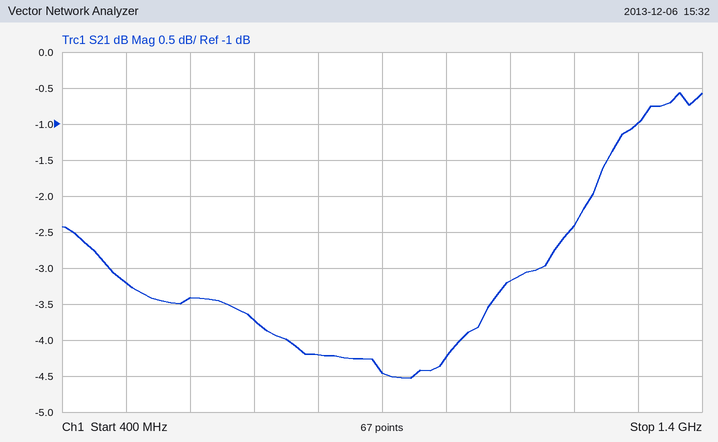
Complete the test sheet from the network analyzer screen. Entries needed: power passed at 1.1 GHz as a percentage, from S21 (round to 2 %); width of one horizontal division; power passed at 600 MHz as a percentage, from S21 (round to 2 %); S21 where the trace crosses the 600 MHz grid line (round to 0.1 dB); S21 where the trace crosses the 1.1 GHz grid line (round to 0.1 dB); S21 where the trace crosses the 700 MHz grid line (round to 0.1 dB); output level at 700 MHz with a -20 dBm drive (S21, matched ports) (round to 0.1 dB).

48 %
100 MHz
46 %
-3.4 dB
-3.2 dB
-3.7 dB
-23.7 dBm
